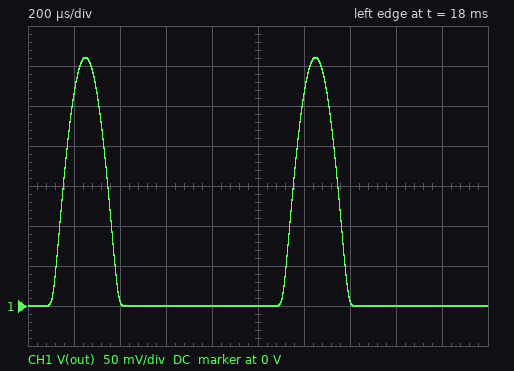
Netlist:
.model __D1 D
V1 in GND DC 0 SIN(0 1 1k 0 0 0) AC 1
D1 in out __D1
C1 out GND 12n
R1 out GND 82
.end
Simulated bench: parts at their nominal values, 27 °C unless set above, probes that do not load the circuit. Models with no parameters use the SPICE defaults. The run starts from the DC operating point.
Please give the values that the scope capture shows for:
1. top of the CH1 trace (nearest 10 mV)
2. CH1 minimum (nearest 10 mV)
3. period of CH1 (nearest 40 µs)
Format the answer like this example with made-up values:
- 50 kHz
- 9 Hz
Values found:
- 310 mV
- 0 V
- 1.00 ms
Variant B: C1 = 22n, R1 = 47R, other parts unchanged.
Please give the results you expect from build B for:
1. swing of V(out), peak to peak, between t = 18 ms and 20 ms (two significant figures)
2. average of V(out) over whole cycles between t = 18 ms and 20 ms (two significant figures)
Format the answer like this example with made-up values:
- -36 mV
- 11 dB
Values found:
- 300 mV
- 53 mV
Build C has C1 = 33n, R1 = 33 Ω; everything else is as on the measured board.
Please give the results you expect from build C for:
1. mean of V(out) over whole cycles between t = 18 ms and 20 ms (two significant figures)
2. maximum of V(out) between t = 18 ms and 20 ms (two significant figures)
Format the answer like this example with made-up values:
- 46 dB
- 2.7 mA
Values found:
- 51 mV
- 290 mV
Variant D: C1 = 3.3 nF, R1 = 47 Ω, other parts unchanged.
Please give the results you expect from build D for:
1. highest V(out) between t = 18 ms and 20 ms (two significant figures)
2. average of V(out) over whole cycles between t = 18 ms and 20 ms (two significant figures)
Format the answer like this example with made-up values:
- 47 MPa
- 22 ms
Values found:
- 300 mV
- 53 mV
